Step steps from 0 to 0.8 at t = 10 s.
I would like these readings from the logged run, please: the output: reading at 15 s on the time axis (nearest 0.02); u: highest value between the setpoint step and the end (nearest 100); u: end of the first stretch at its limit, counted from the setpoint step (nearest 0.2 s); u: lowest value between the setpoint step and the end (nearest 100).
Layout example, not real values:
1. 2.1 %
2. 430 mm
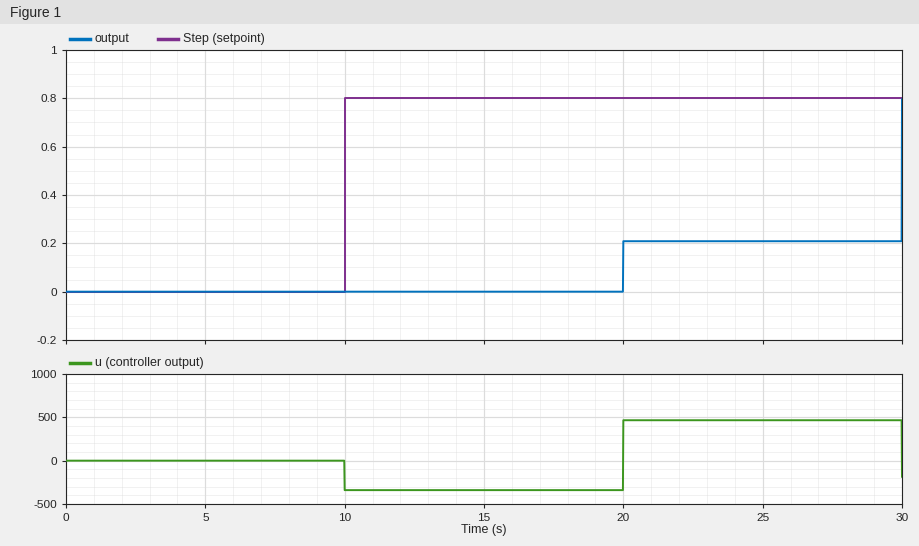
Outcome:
1. 0.00
2. 500
3. 10.0 s
4. -300
